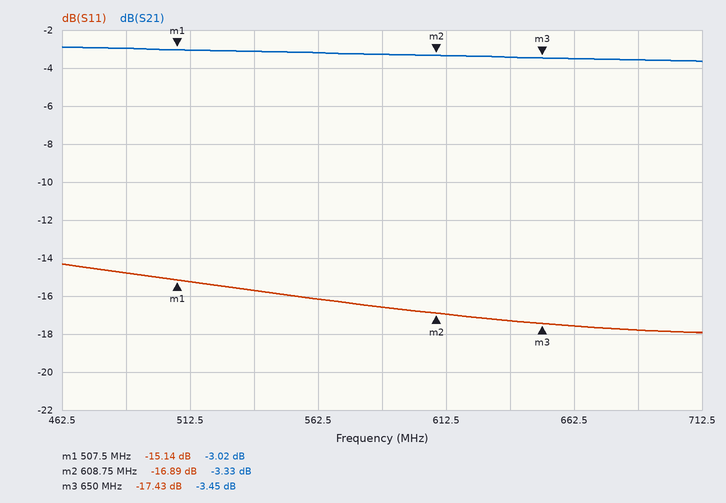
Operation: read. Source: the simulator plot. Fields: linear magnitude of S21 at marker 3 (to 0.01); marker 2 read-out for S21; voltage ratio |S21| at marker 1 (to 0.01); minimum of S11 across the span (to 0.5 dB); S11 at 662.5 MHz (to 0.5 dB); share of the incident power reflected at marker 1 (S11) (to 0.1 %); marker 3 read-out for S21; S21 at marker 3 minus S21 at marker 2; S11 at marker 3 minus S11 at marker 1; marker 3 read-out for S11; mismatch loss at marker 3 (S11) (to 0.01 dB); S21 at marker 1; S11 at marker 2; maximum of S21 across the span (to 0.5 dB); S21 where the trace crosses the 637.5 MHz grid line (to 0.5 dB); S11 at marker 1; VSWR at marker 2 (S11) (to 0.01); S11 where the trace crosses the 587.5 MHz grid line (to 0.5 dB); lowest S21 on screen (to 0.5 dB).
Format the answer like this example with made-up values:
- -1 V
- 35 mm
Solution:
- 0.67
- -3.33 dB
- 0.71
- -18.0 dB
- -17.5 dB
- 3.1 %
- -3.45 dB
- -0.12 dB
- -2.29 dB
- -17.43 dB
- 0.08 dB
- -3.02 dB
- -16.89 dB
- -3.0 dB
- -3.5 dB
- -15.14 dB
- 1.33
- -16.5 dB
- -3.5 dB
